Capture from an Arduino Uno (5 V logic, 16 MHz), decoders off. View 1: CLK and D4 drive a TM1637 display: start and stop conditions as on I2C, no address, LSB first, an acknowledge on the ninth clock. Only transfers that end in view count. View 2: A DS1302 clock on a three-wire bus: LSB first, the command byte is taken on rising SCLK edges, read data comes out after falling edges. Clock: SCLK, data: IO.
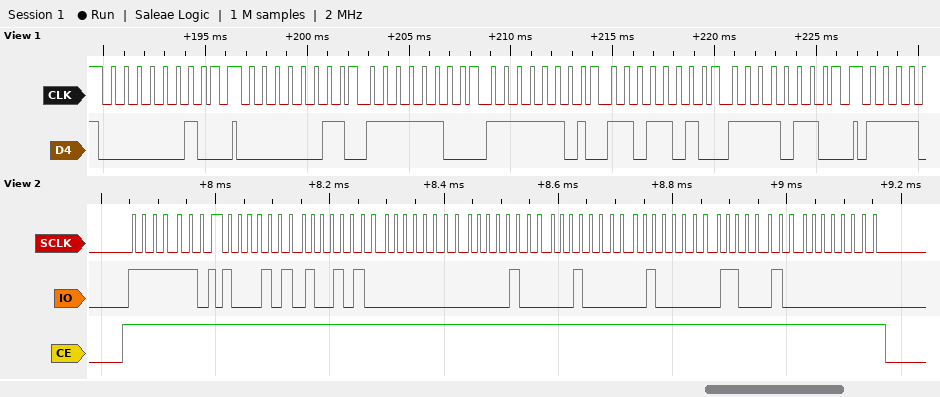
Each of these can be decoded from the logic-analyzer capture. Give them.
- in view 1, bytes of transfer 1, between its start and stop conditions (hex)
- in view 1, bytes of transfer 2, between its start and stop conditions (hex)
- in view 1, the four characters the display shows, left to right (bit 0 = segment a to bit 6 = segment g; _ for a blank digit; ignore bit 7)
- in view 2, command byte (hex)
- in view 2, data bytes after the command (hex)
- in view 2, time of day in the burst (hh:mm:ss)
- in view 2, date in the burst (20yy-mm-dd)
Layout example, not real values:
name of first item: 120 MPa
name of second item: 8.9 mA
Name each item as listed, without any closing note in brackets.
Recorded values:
in view 1, bytes of transfer 1, between its start and stop conditions: 40
in view 1, bytes of transfer 2, between its start and stop conditions: C0 3F BF 5B 6F
in view 1, the four characters the display shows, left to right: 0029
in view 2, command byte: 0xBF
in view 2, data bytes after the command: 51 29 00 10 04 02 23 00
in view 2, time of day in the burst: 00:29:51
in view 2, date in the burst: 2023-04-10
